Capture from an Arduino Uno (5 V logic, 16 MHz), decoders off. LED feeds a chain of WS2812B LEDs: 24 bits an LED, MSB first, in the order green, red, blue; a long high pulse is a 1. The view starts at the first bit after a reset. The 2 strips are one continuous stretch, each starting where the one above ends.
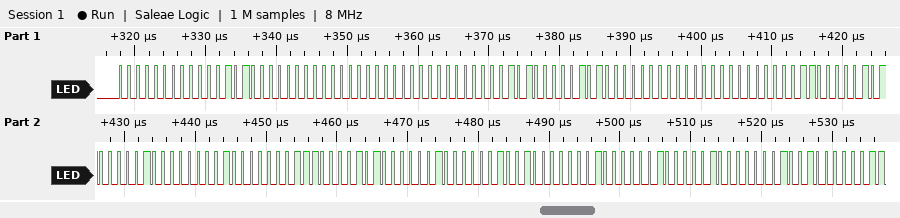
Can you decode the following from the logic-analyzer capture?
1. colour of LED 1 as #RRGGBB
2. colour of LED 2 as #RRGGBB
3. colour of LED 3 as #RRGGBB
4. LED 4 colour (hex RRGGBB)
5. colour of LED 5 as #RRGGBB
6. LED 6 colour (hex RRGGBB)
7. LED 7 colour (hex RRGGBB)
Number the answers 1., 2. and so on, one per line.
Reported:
1. #0A0000
2. #00000A
3. #000A00
4. #0A0608
5. #07040A
6. #090401
7. #080209
